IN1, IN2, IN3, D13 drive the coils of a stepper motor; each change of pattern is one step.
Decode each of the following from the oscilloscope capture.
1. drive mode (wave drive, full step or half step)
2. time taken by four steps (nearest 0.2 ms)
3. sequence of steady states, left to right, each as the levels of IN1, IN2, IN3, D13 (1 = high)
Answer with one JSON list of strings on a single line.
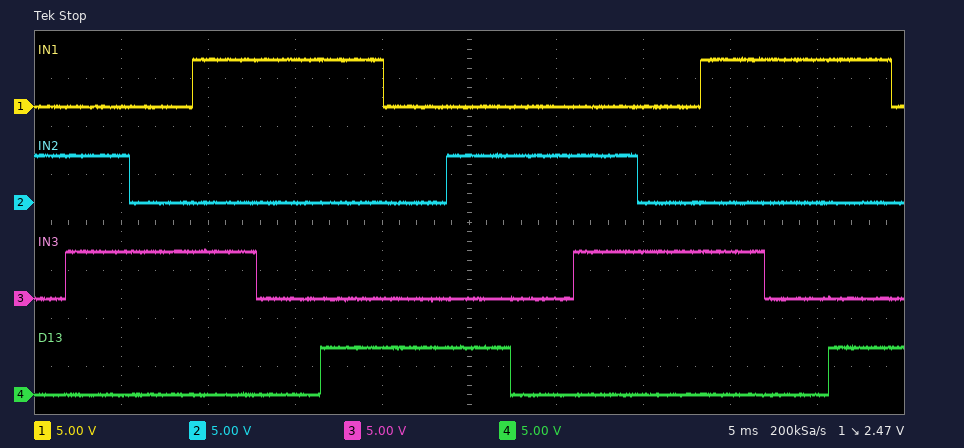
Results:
["half step", "14.6 ms", "0100 0110 0010 1010 1000 1001 0001 0101 0100 0110 0010 1010 1000 1001 0001"]
